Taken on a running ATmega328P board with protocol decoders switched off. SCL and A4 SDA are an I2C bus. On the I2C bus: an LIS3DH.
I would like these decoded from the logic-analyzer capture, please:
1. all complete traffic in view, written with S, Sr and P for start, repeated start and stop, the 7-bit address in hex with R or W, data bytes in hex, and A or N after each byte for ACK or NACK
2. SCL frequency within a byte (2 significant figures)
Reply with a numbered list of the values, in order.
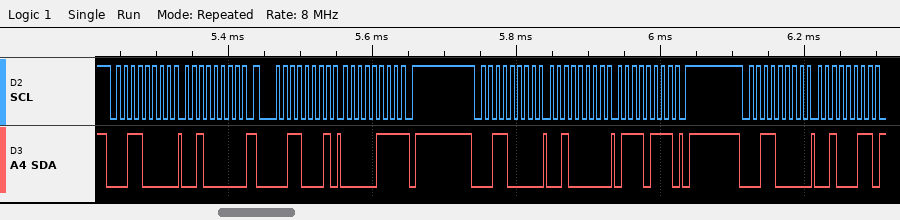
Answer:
1. S 18W A 20 A Sr 18R A 07 N P S 18W A 20 A 77 A P S 18W A 23 A
2. 100 kHz
